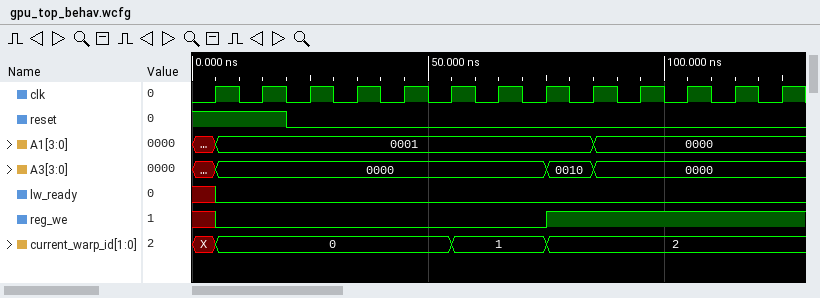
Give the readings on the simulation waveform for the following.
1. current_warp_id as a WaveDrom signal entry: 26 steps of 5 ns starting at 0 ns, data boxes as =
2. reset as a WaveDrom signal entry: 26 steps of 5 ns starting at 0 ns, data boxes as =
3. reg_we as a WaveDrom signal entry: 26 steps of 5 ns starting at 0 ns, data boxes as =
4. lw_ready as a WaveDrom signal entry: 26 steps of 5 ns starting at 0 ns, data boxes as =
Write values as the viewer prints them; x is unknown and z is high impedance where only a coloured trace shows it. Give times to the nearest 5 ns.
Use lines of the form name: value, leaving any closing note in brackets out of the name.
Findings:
current_warp_id as a WaveDrom signal entry: 26 steps of 5 ns starting at 0 ns, data boxes as =: {name: 'current_warp_id', wave: 'x=.........=...=..........', data: '0 1 2'}
reset as a WaveDrom signal entry: 26 steps of 5 ns starting at 0 ns, data boxes as =: {name: 'reset', wave: '1...0.....................'}
reg_we as a WaveDrom signal entry: 26 steps of 5 ns starting at 0 ns, data boxes as =: {name: 'reg_we', wave: 'x0.............1..........'}
lw_ready as a WaveDrom signal entry: 26 steps of 5 ns starting at 0 ns, data boxes as =: {name: 'lw_ready', wave: 'x0........................'}
